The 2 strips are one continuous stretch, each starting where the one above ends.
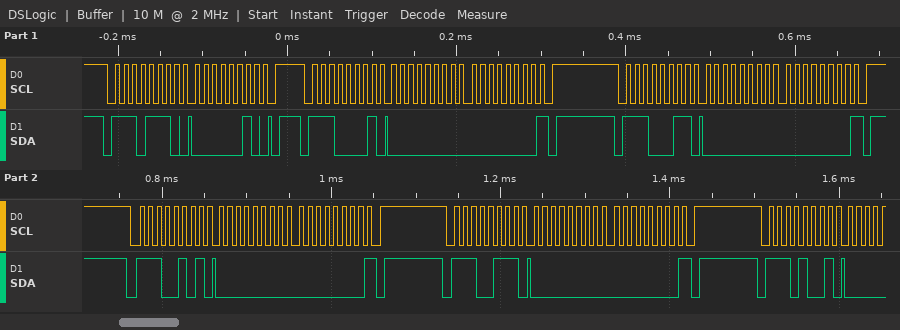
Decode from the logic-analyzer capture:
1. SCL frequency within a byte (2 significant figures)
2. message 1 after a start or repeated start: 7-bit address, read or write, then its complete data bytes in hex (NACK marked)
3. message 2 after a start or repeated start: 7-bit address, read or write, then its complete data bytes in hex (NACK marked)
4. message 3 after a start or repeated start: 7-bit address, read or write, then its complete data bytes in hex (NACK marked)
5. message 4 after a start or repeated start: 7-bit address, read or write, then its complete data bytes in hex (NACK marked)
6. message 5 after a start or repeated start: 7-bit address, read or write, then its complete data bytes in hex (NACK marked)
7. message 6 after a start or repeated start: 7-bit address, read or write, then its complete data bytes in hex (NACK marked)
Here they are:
100 kHz
0x77 write: 02
0x70 read: 00 00 NACK
0x71 read: 00 00 NACK
0x72 read: 00 00 NACK
0x73 read: 00 00 NACK
0x74 read
